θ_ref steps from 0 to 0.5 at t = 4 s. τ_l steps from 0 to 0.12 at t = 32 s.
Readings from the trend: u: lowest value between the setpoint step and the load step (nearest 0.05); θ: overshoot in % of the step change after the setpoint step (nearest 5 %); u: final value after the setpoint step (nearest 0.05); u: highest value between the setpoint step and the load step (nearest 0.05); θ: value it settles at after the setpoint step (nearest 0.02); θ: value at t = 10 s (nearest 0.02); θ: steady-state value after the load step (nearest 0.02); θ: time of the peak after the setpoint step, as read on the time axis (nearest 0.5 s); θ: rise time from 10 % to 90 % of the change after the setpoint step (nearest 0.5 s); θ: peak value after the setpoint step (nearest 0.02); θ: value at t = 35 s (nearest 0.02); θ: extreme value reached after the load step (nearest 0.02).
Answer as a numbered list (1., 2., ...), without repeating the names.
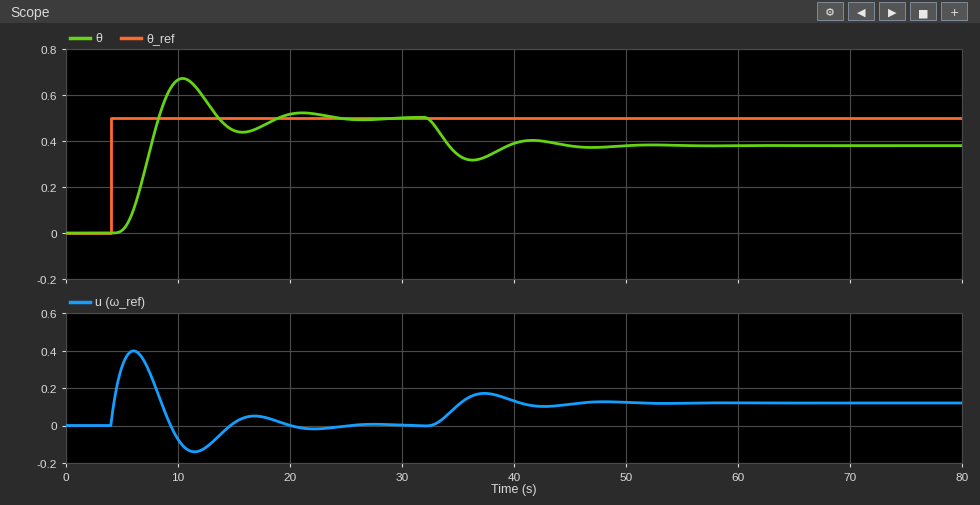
1. -0.15
2. 35 %
3. 0.00
4. 0.40
5. 0.50
6. 0.66
7. 0.38
8. 10.5 s
9. 2.5 s
10. 0.68
11. 0.34
12. 0.32
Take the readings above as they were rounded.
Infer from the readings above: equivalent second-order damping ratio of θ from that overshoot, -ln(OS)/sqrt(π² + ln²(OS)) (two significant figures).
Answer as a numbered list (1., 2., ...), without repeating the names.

1. 0.32
